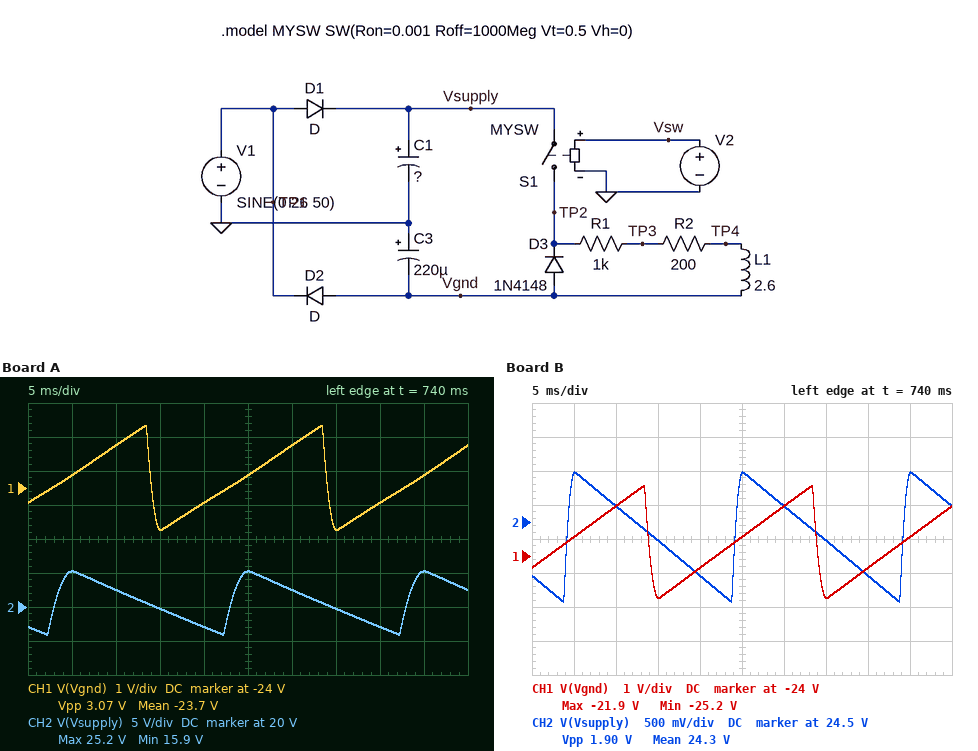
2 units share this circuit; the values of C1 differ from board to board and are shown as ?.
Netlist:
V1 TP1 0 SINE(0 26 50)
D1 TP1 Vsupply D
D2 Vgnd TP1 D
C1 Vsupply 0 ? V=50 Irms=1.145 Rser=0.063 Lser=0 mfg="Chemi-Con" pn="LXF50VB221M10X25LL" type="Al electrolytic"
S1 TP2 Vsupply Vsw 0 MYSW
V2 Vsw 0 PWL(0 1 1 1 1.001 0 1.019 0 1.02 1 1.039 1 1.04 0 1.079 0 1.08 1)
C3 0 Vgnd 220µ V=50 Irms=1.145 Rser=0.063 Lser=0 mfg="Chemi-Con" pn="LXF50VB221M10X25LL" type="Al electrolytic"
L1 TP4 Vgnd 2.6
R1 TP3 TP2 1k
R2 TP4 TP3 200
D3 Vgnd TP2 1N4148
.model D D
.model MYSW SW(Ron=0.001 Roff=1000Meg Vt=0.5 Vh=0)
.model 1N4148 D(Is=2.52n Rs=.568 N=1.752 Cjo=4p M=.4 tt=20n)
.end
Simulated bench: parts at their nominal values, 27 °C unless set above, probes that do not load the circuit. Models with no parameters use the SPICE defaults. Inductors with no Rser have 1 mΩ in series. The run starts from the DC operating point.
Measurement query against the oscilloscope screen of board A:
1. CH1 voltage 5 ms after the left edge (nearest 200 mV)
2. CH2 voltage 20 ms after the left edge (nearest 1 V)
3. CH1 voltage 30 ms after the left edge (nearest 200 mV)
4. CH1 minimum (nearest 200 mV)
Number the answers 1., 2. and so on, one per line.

1. -23.6 V
2. 17 V
3. -22.8 V
4. -25.2 V
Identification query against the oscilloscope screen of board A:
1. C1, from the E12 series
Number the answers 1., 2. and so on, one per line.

1. 68 µF
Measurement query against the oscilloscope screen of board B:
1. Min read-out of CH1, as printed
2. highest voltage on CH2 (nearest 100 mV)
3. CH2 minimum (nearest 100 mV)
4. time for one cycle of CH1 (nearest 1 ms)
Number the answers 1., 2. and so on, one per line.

1. -25.2 V
2. 25.2 V
3. 23.3 V
4. 20 ms
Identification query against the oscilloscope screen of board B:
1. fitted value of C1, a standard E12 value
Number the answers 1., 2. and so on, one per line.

1. 390 µF
